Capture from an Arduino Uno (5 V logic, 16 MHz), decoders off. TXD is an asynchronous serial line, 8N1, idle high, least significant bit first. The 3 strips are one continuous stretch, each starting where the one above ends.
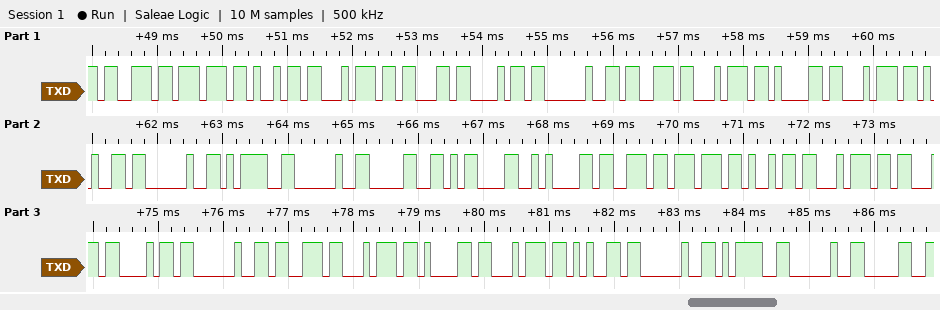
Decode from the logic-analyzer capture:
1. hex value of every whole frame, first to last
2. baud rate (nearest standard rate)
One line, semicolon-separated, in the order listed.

73 77 69 74 63 68 20 73 74 61 74 65 20 3D 20 30 0D 0A 73 77 69 74 63 68 20 73 74 61 74 65 20 3D 20 30; 9600 baud
